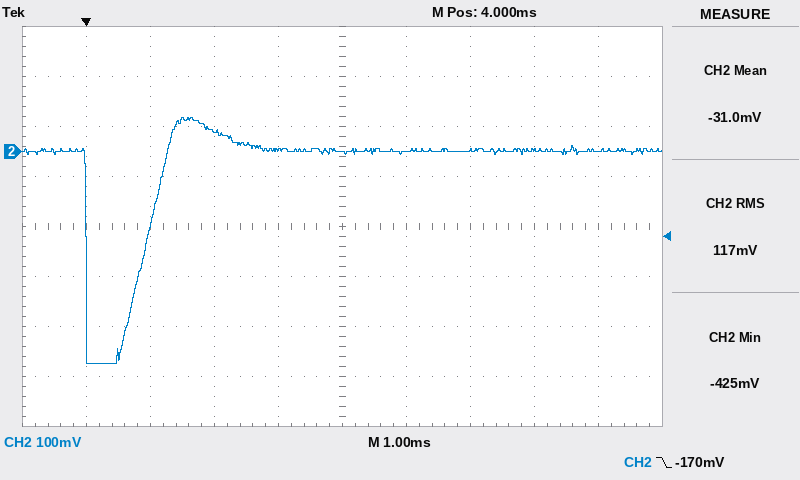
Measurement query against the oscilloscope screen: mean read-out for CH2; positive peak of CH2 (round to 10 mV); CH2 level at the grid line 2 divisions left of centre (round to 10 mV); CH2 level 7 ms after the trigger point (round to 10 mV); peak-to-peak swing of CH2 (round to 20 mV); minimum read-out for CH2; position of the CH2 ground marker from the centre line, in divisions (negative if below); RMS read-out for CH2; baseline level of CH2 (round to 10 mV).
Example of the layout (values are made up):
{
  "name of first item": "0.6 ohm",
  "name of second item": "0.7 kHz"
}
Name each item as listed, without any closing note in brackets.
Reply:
{
  "mean read-out for CH2": "-31.0 mV",
  "positive peak of CH2": "70 mV",
  "CH2 level at the grid line 2 divisions left of centre": "40 mV",
  "CH2 level 7 ms after the trigger point": "0 mV",
  "peak-to-peak swing of CH2": "500 mV",
  "minimum read-out for CH2": "-425 mV",
  "position of the CH2 ground marker from the centre line, in divisions": "+1.5 div",
  "RMS read-out for CH2": "117 mV",
  "baseline level of CH2": "0 mV"
}
